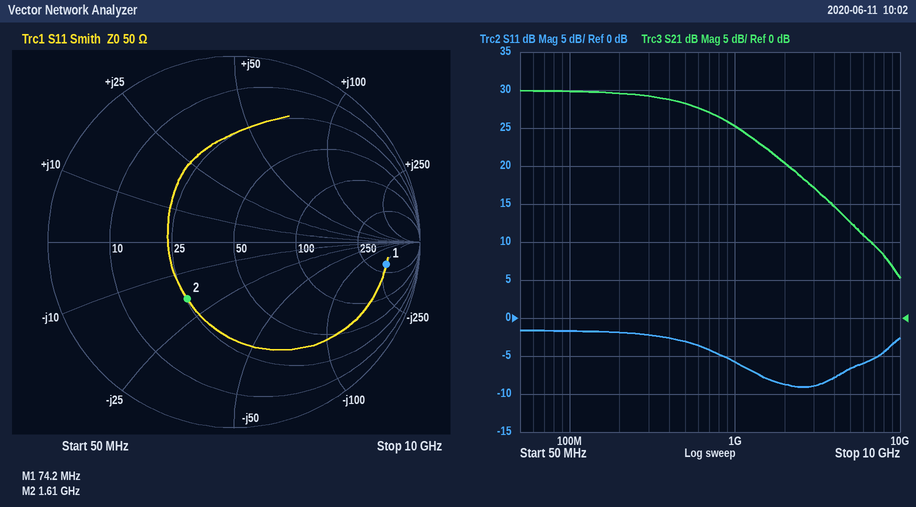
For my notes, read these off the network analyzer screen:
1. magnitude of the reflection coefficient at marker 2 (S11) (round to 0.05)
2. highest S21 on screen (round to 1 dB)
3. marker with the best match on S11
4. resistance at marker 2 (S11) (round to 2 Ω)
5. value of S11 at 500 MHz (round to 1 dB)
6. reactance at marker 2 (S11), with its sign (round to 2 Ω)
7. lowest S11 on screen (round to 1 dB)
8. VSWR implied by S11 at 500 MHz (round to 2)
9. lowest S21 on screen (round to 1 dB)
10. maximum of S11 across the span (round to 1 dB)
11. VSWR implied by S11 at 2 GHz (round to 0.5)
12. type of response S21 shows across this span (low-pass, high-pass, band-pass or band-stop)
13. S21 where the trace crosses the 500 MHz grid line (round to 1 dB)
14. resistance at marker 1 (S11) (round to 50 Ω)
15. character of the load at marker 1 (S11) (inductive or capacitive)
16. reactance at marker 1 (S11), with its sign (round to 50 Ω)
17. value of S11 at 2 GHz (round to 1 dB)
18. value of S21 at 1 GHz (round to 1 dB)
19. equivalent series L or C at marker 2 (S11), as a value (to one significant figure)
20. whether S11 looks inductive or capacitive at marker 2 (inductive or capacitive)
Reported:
0.40
30 dB
marker 2
26 Ω
-3 dB
-18 Ω
-9 dB
6
5 dB
-2 dB
2.0
low-pass
28 dB
350 Ω
capacitive
-250 Ω
-9 dB
25 dB
5 pF
capacitive
